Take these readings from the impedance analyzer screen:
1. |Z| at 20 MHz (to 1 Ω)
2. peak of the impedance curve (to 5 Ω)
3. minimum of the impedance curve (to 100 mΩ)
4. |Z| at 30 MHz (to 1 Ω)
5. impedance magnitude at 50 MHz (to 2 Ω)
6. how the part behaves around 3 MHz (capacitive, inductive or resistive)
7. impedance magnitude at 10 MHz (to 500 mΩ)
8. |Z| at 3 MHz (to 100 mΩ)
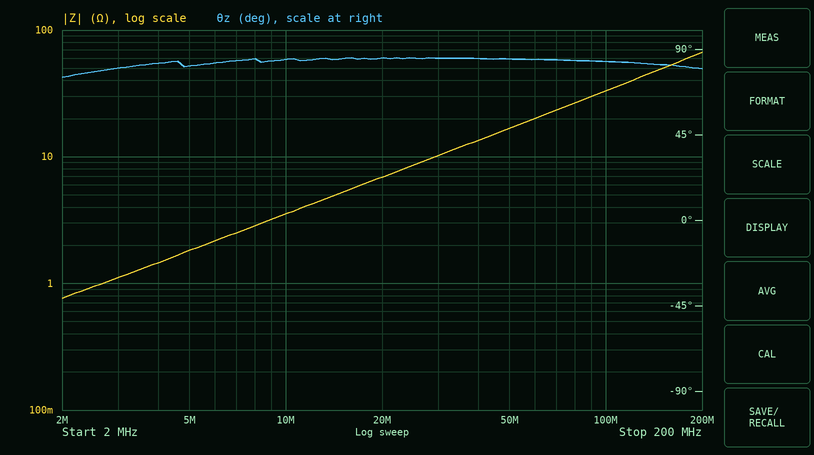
7 Ω
65 Ω
800 mΩ
10 Ω
16 Ω
inductive
3.5 Ω
1.1 Ω
